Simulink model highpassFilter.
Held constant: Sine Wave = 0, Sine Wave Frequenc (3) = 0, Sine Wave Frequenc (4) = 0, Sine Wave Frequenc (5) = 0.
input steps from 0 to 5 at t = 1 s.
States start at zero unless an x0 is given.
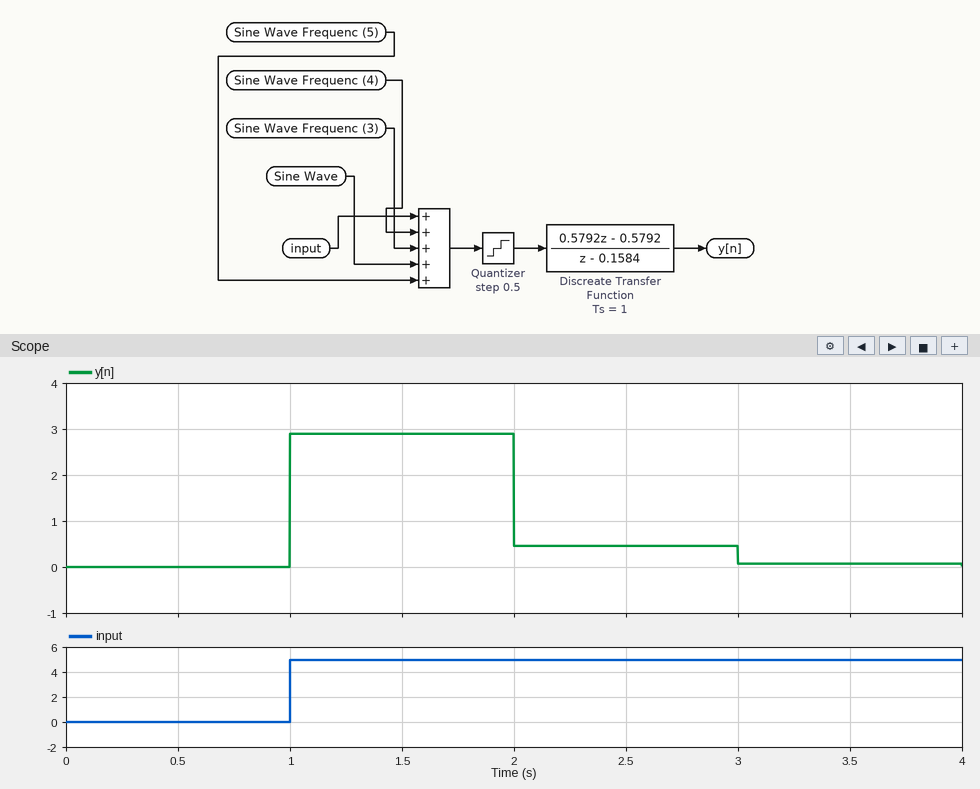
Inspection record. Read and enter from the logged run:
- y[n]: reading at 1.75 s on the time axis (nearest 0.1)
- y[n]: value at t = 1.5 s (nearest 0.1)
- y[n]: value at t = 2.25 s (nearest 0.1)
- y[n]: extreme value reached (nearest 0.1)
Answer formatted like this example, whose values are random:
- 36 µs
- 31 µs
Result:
- 2.9
- 2.9
- 0.5
- 2.9
